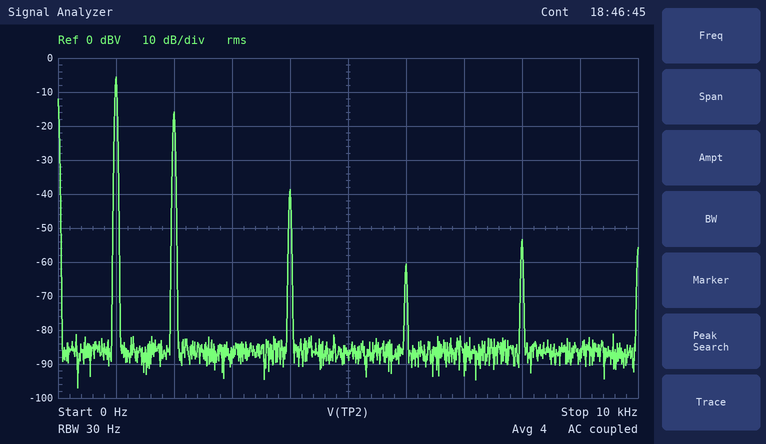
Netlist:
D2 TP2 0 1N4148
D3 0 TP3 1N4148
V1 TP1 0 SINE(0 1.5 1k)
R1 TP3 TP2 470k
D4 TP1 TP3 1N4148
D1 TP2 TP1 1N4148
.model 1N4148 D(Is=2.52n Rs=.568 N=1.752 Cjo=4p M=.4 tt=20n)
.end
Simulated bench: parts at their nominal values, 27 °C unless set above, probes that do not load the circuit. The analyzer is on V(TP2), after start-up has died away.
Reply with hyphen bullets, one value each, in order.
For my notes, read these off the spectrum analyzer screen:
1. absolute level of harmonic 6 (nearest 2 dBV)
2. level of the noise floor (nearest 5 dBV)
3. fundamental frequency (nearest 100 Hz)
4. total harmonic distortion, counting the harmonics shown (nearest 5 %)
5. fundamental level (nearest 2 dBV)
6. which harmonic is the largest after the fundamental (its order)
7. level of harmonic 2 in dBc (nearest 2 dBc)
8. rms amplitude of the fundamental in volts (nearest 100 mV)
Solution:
- -60 dBV
- -85 dBV
- 1.0 kHz
- 30 %
- -6 dBV
- 2
- -10 dBc
- 500 mV
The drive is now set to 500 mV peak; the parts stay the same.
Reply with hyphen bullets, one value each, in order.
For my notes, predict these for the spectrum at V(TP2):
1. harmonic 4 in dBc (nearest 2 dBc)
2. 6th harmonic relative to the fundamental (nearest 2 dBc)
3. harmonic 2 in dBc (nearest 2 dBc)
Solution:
- -38 dBc
- -54 dBc
- -20 dBc
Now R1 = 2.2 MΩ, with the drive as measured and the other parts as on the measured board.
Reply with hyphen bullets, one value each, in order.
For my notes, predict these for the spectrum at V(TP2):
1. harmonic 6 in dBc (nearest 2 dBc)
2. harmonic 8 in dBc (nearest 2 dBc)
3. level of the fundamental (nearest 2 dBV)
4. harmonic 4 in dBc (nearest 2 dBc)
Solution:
- -42 dBc
- -54 dBc
- -6 dBV
- -28 dBc
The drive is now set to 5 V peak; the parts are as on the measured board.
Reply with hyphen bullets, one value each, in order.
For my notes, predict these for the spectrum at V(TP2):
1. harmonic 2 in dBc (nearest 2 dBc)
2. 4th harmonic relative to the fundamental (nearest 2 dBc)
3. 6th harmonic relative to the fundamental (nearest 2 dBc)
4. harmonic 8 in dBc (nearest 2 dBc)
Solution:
- -8 dBc
- -24 dBc
- -32 dBc
- -40 dBc
